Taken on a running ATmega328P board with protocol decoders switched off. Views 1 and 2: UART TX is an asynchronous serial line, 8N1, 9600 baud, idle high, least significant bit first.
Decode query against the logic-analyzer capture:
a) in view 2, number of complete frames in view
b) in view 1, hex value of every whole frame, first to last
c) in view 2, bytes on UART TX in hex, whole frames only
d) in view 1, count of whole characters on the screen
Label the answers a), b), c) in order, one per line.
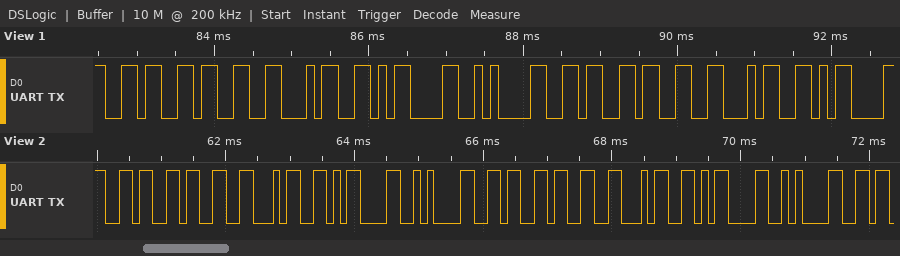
a) 10
b) 36 33 34 0D 0A 36 33 34 0D
c) 36 33 34 0D 0A 36 33 34 0D 0A
d) 9
